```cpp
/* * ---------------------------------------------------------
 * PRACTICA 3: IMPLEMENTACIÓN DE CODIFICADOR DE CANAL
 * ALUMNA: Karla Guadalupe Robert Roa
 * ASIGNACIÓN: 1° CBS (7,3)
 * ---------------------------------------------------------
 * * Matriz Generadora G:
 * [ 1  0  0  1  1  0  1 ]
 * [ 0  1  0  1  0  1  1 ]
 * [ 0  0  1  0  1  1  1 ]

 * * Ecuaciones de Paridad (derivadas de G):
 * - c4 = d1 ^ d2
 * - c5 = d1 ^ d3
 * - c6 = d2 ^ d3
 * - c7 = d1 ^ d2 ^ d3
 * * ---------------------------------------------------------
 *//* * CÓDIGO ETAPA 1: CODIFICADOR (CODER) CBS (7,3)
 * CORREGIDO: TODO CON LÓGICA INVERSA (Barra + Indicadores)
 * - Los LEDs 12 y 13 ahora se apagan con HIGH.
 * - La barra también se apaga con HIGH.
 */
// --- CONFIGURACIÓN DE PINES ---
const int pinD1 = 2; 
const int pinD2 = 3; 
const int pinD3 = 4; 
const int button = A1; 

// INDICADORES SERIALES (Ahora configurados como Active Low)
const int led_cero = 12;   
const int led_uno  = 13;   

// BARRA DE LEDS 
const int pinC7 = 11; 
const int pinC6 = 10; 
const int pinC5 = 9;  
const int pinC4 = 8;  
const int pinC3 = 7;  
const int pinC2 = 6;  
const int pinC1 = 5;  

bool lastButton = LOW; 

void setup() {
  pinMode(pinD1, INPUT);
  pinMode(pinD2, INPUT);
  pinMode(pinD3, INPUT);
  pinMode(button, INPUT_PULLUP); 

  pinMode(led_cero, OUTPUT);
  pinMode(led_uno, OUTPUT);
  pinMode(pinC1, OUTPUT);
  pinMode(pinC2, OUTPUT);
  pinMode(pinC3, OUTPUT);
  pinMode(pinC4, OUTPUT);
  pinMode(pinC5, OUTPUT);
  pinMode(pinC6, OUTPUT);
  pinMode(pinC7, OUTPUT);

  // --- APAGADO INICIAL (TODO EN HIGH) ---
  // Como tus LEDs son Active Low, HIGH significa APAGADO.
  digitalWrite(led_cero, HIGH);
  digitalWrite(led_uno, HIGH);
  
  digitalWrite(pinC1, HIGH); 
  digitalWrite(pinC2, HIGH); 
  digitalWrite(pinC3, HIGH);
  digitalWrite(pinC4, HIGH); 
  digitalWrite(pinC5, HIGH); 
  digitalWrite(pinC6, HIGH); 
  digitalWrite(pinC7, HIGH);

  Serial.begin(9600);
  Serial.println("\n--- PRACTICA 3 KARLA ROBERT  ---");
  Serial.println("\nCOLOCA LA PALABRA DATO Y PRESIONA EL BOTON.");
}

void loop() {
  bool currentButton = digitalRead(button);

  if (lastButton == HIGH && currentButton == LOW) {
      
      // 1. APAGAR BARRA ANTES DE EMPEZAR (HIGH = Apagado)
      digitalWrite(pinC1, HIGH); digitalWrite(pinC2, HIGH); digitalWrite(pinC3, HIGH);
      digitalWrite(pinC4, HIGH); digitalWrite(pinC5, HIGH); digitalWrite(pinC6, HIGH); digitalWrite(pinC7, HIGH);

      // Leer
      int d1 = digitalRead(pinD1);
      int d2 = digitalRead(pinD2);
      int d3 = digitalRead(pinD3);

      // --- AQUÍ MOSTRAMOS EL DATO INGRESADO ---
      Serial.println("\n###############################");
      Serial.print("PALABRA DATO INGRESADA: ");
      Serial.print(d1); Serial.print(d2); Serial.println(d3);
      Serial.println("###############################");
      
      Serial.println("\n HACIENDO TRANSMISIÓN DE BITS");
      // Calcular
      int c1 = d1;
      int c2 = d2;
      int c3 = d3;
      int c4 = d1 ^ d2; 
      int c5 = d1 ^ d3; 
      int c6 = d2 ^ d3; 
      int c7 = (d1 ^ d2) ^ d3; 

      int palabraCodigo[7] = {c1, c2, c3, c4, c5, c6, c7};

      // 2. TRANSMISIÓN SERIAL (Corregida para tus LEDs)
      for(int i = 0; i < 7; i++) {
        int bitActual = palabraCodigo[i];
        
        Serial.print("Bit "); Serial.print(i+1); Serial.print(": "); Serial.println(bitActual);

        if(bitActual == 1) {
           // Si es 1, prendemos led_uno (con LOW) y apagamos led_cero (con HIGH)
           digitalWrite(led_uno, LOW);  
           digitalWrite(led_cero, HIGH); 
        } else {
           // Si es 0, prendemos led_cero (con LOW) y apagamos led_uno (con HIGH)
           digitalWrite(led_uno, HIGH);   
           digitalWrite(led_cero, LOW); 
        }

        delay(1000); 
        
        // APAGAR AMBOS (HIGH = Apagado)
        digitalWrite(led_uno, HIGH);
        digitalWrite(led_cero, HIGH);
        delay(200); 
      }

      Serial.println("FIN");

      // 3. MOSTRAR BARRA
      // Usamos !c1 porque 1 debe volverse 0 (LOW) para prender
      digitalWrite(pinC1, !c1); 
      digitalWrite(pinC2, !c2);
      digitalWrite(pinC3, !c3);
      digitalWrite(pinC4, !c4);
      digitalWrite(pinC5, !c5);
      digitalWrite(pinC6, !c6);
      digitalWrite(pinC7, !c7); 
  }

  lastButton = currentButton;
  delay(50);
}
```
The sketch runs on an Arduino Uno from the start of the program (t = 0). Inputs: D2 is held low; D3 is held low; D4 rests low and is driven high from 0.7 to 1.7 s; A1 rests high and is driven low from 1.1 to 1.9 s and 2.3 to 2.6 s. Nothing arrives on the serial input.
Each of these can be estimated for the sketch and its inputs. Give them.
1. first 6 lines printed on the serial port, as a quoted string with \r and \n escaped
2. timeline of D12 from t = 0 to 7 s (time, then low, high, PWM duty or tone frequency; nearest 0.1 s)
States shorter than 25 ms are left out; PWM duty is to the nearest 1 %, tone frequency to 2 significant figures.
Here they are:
"\n--- PRACTICA 3 KARLA ROBERT  ---\r\n\nCOLOCA LA PALABRA DATO Y PRESIONA EL BOTON.\r\n\n###############################\r\n"
0 s high; 1.2 s low; 2.2 s high; 2.4 s low; 3.4 s high; 4.8 s low; 5.8 s high
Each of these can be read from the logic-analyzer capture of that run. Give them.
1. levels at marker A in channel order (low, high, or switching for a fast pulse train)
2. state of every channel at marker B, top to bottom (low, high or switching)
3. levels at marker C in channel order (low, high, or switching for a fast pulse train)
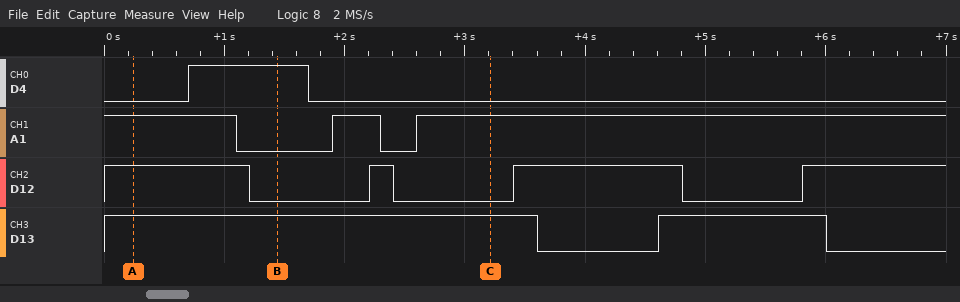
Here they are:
D4 low, A1 high, D12 high, D13 high
D4 high, A1 low, D12 low, D13 high
D4 low, A1 high, D12 low, D13 high
